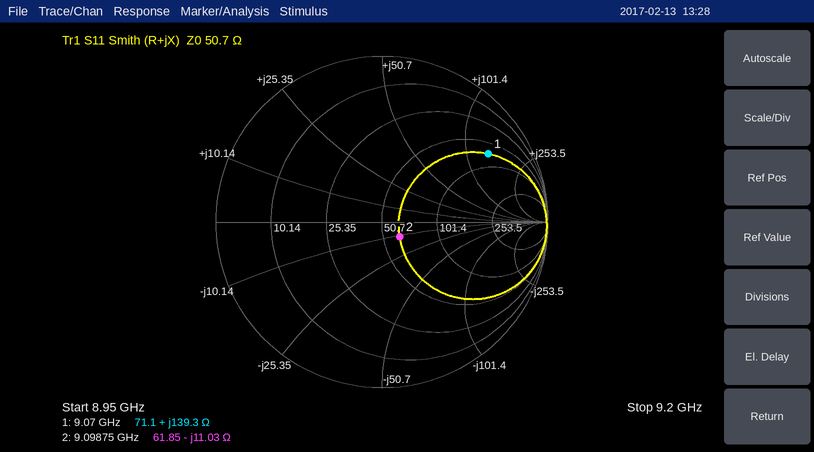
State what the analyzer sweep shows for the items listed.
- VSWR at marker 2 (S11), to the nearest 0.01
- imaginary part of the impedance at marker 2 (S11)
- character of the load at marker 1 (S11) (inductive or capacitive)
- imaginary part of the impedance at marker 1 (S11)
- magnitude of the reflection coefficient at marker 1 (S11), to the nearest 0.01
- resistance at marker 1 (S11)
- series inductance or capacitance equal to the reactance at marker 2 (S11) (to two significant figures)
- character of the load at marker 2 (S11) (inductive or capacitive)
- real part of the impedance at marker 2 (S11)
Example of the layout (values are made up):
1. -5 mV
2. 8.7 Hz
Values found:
1. 1.32
2. -11.03 Ω
3. inductive
4. +139.3 Ω
5. 0.76
6. 71.1 Ω
7. 1.6 pF
8. capacitive
9. 61.85 Ω
